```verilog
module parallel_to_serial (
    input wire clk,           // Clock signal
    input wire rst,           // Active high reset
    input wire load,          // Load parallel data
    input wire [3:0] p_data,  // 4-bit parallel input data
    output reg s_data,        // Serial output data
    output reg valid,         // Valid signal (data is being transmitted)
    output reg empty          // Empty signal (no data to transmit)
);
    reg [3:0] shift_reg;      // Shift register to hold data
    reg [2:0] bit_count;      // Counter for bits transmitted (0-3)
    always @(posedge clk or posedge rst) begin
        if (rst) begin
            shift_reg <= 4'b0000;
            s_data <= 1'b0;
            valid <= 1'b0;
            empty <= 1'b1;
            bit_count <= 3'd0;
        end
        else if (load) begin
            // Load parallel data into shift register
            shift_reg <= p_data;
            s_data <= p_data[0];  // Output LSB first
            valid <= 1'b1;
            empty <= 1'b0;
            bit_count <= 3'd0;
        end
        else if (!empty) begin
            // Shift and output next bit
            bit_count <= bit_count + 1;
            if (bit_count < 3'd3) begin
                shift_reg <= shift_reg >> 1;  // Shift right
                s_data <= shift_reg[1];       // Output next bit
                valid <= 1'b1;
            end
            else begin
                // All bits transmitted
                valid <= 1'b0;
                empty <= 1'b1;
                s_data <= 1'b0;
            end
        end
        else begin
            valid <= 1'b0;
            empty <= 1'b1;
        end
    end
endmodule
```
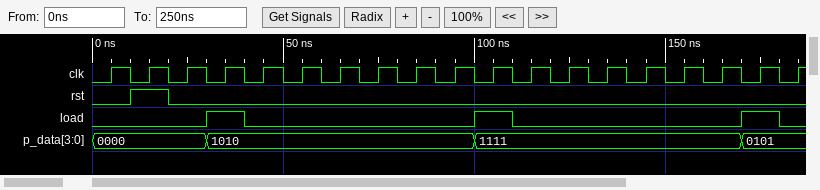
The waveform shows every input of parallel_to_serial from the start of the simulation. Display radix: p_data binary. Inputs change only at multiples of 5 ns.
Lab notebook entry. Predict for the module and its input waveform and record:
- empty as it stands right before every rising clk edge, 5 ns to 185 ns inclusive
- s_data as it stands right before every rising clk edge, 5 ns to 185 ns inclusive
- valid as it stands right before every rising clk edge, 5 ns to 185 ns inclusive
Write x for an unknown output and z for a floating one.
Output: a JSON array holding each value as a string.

["x 1 1 1 0 0 0 0 1 1 1 0 0 0 0 1 1 1 0", "x 0 0 0 0 1 0 1 0 0 0 1 1 1 1 0 0 0 1", "x 0 0 0 1 1 1 1 0 0 0 1 1 1 1 0 0 0 1"]
